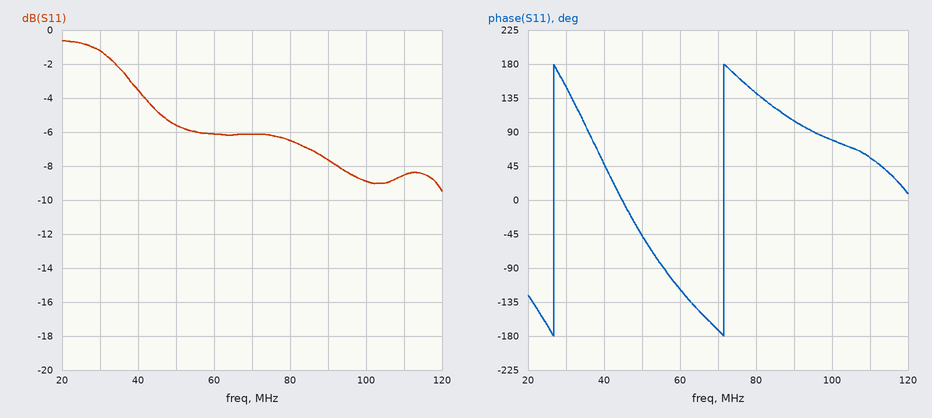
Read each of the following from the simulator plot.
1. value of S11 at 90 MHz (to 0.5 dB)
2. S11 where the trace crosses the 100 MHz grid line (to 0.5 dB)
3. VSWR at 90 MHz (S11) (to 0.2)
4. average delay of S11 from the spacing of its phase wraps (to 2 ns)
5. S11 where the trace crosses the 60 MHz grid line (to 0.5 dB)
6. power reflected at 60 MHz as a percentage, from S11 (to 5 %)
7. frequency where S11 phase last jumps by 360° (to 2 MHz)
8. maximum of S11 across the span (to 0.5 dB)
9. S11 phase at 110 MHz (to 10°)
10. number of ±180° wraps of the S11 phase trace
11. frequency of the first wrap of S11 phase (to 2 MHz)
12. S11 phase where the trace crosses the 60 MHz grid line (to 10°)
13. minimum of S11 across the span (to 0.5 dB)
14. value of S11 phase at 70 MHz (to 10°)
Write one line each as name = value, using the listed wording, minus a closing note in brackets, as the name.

value of S11 at 90 MHz = -7.5 dB
S11 where the trace crosses the 100 MHz grid line = -9.0 dB
VSWR at 90 MHz (S11) = 2.4
average delay of S11 from the spacing of its phase wraps = 22 ns
S11 where the trace crosses the 60 MHz grid line = -6.0 dB
power reflected at 60 MHz as a percentage, from S11 = 25 %
frequency where S11 phase last jumps by 360° = 72 MHz
maximum of S11 across the span = -0.5 dB
S11 phase at 110 MHz = 60°
number of ±180° wraps of the S11 phase trace = 2
frequency of the first wrap of S11 phase = 26 MHz
S11 phase where the trace crosses the 60 MHz grid line = -120°
minimum of S11 across the span = -9.5 dB
value of S11 phase at 70 MHz = -170°
